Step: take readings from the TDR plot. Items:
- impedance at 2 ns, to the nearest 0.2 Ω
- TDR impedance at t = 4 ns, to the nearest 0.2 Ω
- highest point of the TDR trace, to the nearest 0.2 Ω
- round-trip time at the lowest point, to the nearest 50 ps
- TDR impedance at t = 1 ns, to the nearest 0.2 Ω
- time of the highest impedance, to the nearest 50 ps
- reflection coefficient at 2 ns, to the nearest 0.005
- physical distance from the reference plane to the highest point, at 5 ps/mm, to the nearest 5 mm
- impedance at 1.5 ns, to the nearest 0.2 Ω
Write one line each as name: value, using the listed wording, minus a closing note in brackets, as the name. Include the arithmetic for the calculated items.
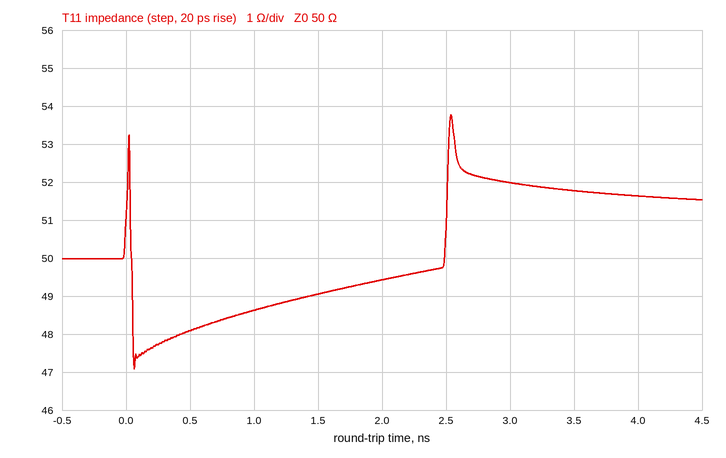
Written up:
impedance at 2 ns, to the nearest 0.2 Ω: 49.4 Ω
TDR impedance at t = 4 ns, to the nearest 0.2 Ω: 51.6 Ω
highest point of the TDR trace, to the nearest 0.2 Ω: 53.8 Ω
round-trip time at the lowest point, to the nearest 50 ps: 50 ps
TDR impedance at t = 1 ns, to the nearest 0.2 Ω: 48.6 Ω
time of the highest impedance, to the nearest 50 ps: 2.55 ns
reflection coefficient at 2 ns, to the nearest 0.005: (49.4 − 50)/(49.4 + 50) ≈ -0.00604, so -0.005 to the nearest 0.005
physical distance from the reference plane to the highest point, at 5 ps/mm, to the nearest 5 mm: 2.55 ns / 2 / 5 ps/mm ≈ 255 mm
impedance at 1.5 ns, to the nearest 0.2 Ω: 49.0 Ω
